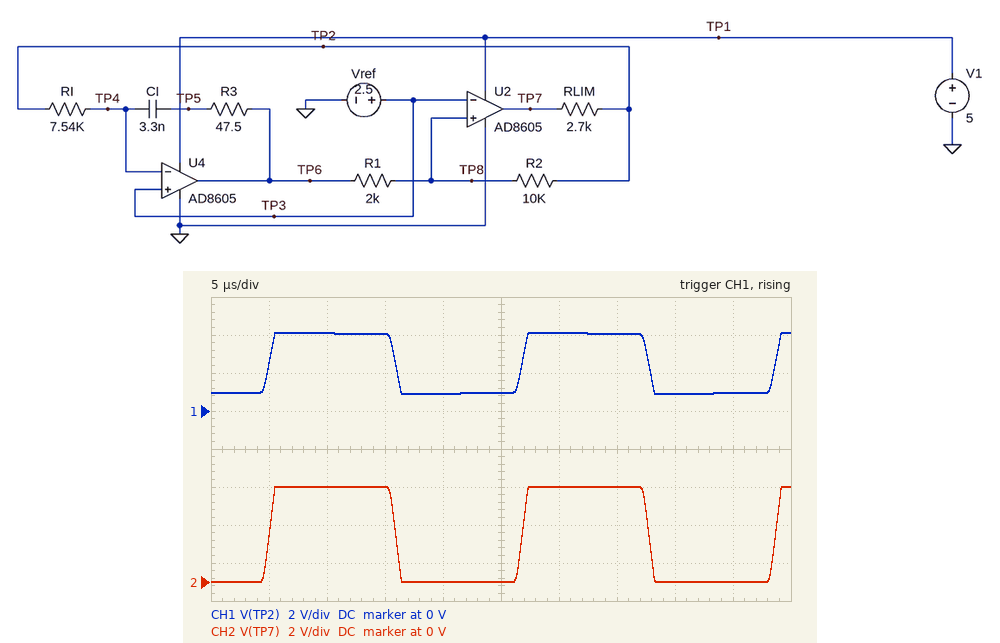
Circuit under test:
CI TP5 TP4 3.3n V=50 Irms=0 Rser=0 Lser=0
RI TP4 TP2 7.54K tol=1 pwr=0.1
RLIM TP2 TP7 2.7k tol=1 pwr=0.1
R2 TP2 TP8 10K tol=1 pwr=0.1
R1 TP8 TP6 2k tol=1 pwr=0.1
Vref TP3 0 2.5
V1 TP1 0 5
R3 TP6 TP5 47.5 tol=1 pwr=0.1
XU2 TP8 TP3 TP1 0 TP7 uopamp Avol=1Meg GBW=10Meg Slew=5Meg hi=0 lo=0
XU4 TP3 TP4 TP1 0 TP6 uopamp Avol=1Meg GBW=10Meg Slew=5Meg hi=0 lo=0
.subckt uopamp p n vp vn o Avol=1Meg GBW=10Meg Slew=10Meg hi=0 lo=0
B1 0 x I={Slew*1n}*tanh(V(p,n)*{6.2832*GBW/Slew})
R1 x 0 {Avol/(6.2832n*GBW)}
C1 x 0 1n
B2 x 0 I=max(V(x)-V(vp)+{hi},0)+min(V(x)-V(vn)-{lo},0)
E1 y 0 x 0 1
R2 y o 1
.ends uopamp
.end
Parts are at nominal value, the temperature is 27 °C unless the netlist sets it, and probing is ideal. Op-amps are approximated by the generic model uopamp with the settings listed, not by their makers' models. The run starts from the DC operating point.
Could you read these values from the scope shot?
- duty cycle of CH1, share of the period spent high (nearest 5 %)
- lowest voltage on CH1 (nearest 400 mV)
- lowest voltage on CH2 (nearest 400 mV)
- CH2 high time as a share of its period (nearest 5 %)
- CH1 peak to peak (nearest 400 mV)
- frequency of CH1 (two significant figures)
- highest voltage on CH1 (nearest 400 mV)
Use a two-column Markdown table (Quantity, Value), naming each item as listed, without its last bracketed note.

| Quantity | Value |
|---|---|
| duty cycle of CH1, share of the period spent high | 50 % |
| lowest voltage on CH1 | 800 mV |
| lowest voltage on CH2 | 0 V |
| CH2 high time as a share of its period | 50 % |
| CH1 peak to peak | 3.2 V |
| frequency of CH1 | 46 kHz |
| highest voltage on CH1 | 4.0 V |
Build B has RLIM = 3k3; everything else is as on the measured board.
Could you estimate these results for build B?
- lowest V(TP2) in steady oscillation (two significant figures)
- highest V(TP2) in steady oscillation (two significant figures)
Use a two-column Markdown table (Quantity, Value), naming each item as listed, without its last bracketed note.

| Quantity | Value |
|---|---|
| lowest V(TP2) in steady oscillation | 990 mV |
| highest V(TP2) in steady oscillation | 4.0 V |
